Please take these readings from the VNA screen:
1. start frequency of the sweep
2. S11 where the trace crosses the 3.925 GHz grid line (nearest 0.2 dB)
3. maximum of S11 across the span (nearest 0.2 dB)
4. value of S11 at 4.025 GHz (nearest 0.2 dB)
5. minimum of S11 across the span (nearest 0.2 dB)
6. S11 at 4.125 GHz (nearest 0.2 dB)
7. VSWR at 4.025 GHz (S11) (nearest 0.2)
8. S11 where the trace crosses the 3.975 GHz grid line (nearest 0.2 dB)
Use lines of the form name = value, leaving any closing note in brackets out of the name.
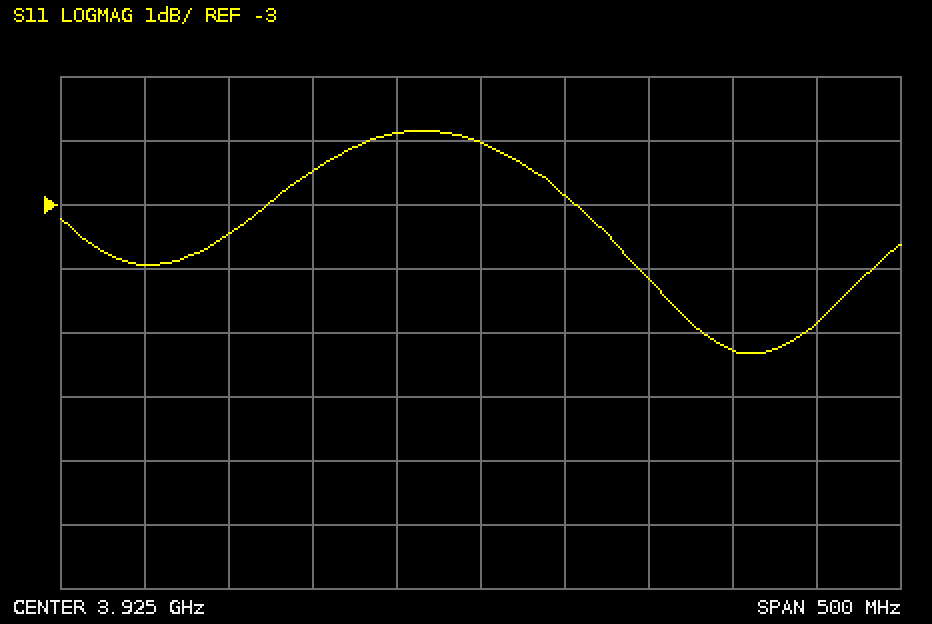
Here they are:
start frequency of the sweep = 3.675 GHz
S11 where the trace crosses the 3.925 GHz grid line = -2.0 dB
maximum of S11 across the span = -1.8 dB
value of S11 at 4.025 GHz = -4.2 dB
minimum of S11 across the span = -5.4 dB
S11 at 4.125 GHz = -4.8 dB
VSWR at 4.025 GHz (S11) = 4.2
S11 where the trace crosses the 3.975 GHz grid line = -2.8 dB
